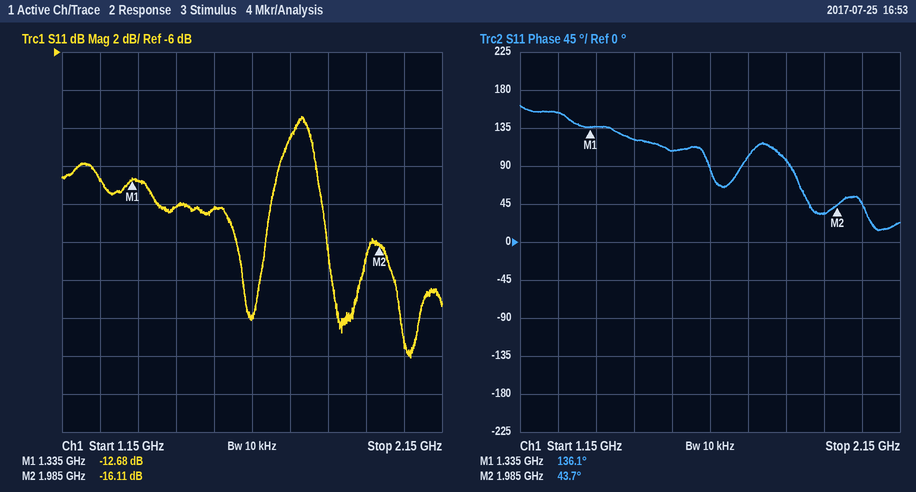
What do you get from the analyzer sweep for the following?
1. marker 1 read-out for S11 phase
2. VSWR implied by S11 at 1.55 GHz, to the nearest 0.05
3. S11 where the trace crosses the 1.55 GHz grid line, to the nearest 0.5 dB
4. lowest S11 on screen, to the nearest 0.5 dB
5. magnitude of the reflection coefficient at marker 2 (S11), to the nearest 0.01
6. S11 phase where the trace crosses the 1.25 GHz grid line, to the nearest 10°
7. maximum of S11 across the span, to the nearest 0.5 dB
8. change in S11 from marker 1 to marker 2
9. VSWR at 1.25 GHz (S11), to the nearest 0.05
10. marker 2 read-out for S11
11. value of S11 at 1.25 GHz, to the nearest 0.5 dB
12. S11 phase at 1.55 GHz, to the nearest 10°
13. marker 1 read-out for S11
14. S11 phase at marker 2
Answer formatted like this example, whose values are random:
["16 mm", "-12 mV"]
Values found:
["136.1°", "1.50", "-14.0 dB", "-22.0 dB", "0.16", "150°", "-9.5 dB", "-3.43 dB", "1.60", "-16.11 dB", "-12.5 dB", "110°", "-12.68 dB", "43.7°"]
